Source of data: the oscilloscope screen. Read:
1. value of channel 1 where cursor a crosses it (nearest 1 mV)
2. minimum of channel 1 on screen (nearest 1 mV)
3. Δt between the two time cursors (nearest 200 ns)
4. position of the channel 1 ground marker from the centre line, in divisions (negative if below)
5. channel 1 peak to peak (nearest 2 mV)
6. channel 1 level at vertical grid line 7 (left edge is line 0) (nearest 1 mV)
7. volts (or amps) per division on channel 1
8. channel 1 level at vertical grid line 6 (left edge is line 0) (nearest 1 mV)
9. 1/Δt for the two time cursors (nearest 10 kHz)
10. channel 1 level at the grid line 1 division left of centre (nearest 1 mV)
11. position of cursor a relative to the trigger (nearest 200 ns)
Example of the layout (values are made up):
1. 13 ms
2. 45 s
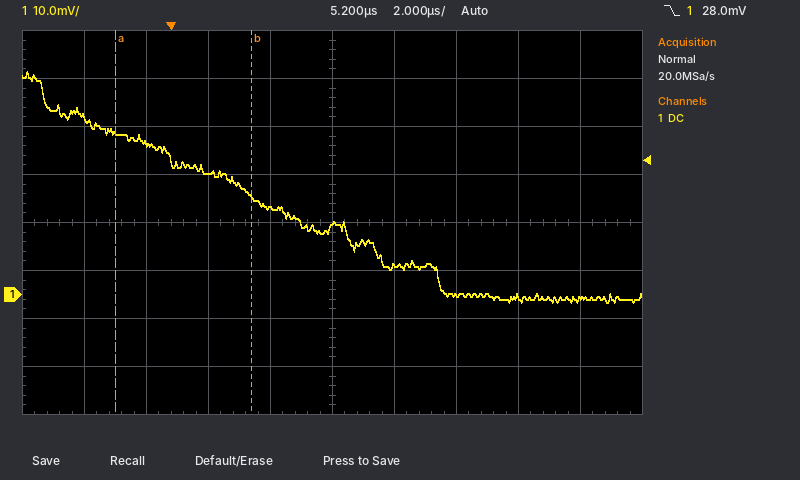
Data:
1. 34 mV
2. -2 mV
3. 4.4 µs
4. -1.5 div
5. 48 mV
6. 0 mV
7. 10 mV
8. 6 mV
9. 230 kHz
10. 18 mV
11. -1.8 µs
